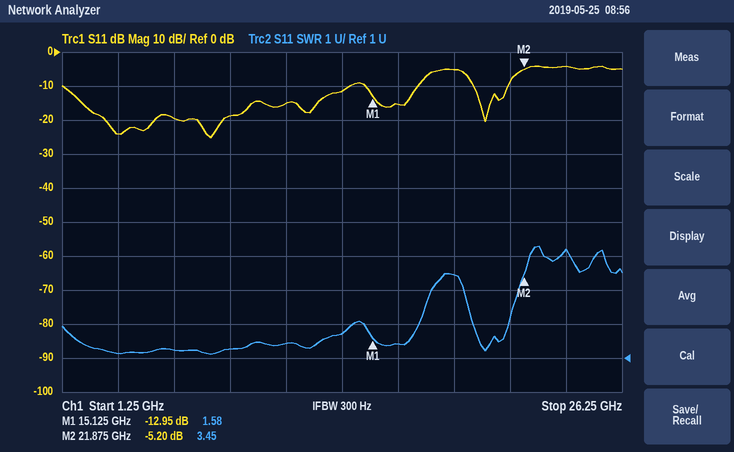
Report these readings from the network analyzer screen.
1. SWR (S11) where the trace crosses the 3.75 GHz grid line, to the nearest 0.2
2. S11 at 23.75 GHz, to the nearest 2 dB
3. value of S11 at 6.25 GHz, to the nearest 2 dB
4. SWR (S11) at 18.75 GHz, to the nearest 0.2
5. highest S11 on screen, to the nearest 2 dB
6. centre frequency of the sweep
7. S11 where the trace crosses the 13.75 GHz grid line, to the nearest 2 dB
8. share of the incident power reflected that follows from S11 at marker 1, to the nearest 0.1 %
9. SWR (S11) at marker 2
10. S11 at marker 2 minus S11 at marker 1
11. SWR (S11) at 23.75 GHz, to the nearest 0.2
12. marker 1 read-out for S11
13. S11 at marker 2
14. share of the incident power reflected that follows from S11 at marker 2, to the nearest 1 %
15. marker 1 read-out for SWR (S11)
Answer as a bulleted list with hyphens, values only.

- 1.2
- -4 dB
- -20 dB
- 3.4
- -4 dB
- 13.75 GHz
- -12 dB
- 5.1 %
- 3.45
- 7.75 dB
- 4.2
- -12.95 dB
- -5.20 dB
- 30 %
- 1.58
